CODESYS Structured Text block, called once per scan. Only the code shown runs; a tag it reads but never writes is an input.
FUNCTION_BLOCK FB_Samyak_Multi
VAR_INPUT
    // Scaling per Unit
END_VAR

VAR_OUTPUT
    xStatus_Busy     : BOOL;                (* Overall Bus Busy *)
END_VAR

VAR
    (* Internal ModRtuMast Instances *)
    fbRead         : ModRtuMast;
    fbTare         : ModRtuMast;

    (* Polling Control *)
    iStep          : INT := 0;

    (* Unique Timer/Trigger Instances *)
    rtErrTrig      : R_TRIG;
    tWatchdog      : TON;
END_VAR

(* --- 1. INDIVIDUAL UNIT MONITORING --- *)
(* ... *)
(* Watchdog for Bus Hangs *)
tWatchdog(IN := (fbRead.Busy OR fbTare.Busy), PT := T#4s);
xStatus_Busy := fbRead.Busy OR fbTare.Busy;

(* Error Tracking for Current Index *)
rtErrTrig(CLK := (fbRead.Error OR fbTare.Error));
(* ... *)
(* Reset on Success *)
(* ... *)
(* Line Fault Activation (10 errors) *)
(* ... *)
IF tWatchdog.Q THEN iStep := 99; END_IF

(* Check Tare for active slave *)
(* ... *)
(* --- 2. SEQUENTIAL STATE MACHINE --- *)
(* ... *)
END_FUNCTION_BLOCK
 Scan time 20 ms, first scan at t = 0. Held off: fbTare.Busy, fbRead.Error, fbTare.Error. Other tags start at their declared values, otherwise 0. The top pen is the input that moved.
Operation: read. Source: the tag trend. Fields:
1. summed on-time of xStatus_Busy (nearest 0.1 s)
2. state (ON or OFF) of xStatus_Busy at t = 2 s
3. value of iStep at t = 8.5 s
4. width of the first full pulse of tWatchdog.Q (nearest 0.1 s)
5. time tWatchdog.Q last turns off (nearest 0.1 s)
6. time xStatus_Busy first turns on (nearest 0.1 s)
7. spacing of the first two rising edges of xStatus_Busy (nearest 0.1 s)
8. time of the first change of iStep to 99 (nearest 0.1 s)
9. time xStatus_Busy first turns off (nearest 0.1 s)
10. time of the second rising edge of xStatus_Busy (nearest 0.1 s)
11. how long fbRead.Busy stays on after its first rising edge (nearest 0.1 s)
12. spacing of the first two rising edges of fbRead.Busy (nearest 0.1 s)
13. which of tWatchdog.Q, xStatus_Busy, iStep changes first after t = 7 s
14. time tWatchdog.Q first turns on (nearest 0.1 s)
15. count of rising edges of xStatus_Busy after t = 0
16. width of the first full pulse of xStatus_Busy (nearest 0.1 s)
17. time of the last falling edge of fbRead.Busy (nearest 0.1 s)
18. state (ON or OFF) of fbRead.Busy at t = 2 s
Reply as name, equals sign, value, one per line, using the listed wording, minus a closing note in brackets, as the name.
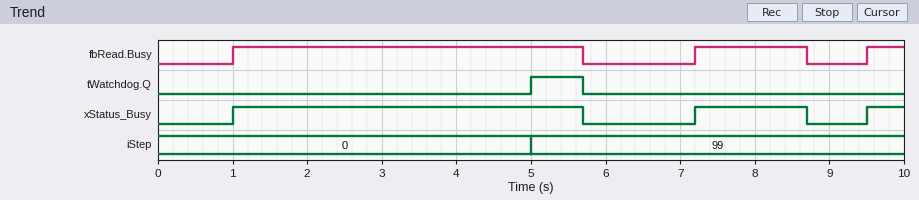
summed on-time of xStatus_Busy = 6.7 s
state (ON or OFF) of xStatus_Busy at t = 2 s = ON
value of iStep at t = 8.5 s = 99
width of the first full pulse of tWatchdog.Q = 0.7 s
time tWatchdog.Q last turns off = 5.7 s
time xStatus_Busy first turns on = 1.0 s
spacing of the first two rising edges of xStatus_Busy = 6.2 s
time of the first change of iStep to 99 = 5.0 s
time xStatus_Busy first turns off = 5.7 s
time of the second rising edge of xStatus_Busy = 7.2 s
how long fbRead.Busy stays on after its first rising edge = 4.7 s
spacing of the first two rising edges of fbRead.Busy = 6.2 s
which of tWatchdog.Q, xStatus_Busy, iStep changes first after t = 7 s = xStatus_Busy
time tWatchdog.Q first turns on = 5.0 s
count of rising edges of xStatus_Busy after t = 0 = 3
width of the first full pulse of xStatus_Busy = 4.7 s
time of the last falling edge of fbRead.Busy = 8.7 s
state (ON or OFF) of fbRead.Busy at t = 2 s = ON
